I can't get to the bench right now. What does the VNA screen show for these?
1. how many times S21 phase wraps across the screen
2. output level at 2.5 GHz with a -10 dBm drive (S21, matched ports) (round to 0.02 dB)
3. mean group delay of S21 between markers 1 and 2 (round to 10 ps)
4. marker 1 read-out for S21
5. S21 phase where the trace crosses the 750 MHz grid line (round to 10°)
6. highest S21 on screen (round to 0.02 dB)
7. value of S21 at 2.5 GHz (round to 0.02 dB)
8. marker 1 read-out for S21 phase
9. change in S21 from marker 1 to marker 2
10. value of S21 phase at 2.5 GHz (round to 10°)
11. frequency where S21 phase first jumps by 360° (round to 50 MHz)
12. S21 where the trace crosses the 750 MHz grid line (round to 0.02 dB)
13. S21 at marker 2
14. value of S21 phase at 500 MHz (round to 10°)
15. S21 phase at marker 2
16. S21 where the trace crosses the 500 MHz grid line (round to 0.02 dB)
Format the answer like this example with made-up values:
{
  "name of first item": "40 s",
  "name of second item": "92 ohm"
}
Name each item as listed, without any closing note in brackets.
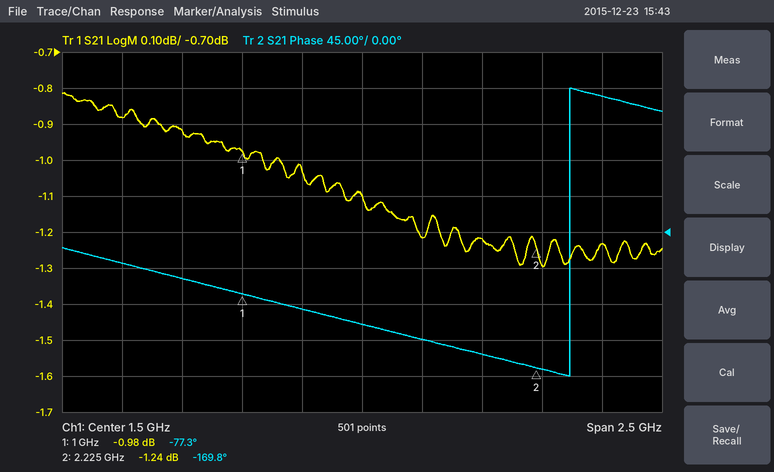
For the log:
{
  "how many times S21 phase wraps across the screen": "1",
  "output level at 2.5 GHz with a -10 dBm drive (S21, matched ports)": "-11.24 dBm",
  "mean group delay of S21 between markers 1 and 2": "210 ps",
  "marker 1 read-out for S21": "-0.98 dB",
  "S21 phase where the trace crosses the 750 MHz grid line": "-60°",
  "highest S21 on screen": "-0.82 dB",
  "value of S21 at 2.5 GHz": "-1.24 dB",
  "marker 1 read-out for S21 phase": "-77.3°",
  "change in S21 from marker 1 to marker 2": "-0.26 dB",
  "value of S21 phase at 2.5 GHz": "170°",
  "frequency where S21 phase first jumps by 360°": "2.35 GHz",
  "S21 where the trace crosses the 750 MHz grid line": "-0.92 dB",
  "S21 at marker 2": "-1.24 dB",
  "value of S21 phase at 500 MHz": "-40°",
  "S21 phase at marker 2": "-169.8°",
  "S21 where the trace crosses the 500 MHz grid line": "-0.88 dB"
}
